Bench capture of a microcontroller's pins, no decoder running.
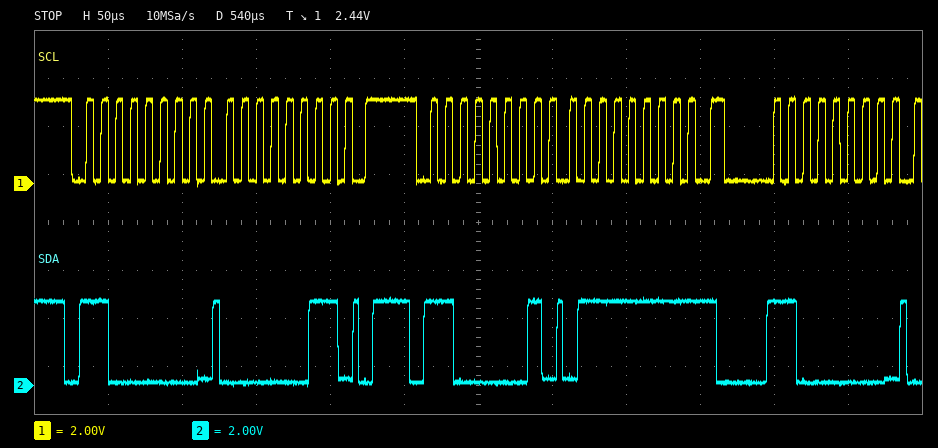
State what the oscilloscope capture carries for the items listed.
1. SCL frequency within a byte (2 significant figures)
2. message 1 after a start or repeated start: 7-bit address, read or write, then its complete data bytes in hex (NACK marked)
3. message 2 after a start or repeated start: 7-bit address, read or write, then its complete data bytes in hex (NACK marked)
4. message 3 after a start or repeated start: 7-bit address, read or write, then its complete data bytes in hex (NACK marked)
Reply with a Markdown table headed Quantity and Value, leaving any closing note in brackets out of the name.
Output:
| Quantity | Value |
|---|---|
| SCL frequency within a byte | 100 kHz |
| message 1 after a start or repeated start: 7-bit address, read or write, then its complete data bytes in hex | 0x60 write: 03 |
| message 2 after a start or repeated start: 7-bit address, read or write, then its complete data bytes in hex | 0x60 read: 7F NACK |
| message 3 after a start or repeated start: 7-bit address, read or write, then its complete data bytes in hex | 0x60 write |
